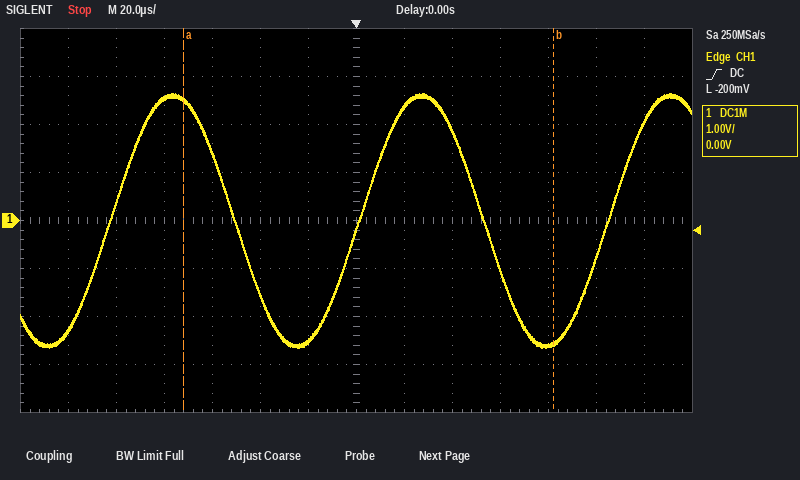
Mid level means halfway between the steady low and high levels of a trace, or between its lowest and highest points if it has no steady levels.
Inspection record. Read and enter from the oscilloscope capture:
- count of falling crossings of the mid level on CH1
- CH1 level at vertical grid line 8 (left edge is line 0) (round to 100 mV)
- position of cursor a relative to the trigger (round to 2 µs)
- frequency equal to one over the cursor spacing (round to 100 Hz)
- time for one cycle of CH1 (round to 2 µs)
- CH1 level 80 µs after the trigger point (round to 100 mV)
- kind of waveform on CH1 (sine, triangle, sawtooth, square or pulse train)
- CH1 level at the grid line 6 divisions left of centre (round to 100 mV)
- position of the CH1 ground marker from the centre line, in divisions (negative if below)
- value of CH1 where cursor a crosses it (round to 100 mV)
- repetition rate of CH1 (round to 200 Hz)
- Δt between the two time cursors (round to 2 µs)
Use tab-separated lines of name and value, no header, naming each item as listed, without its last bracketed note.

count of falling crossings of the mid level on CH1	2
CH1 level at vertical grid line 8 (left edge is line 0)	2.4 V
position of cursor a relative to the trigger	-72 µs
frequency equal to one over the cursor spacing	6.5 kHz
time for one cycle of CH1	104 µs
CH1 level 80 µs after the trigger point	-2.6 V
kind of waveform on CH1	sine
CH1 level at the grid line 6 divisions left of centre	-2.3 V
position of the CH1 ground marker from the centre line, in divisions	0.0 div
value of CH1 where cursor a crosses it	2.5 V
repetition rate of CH1	9.6 kHz
Δt between the two time cursors	154 µs
